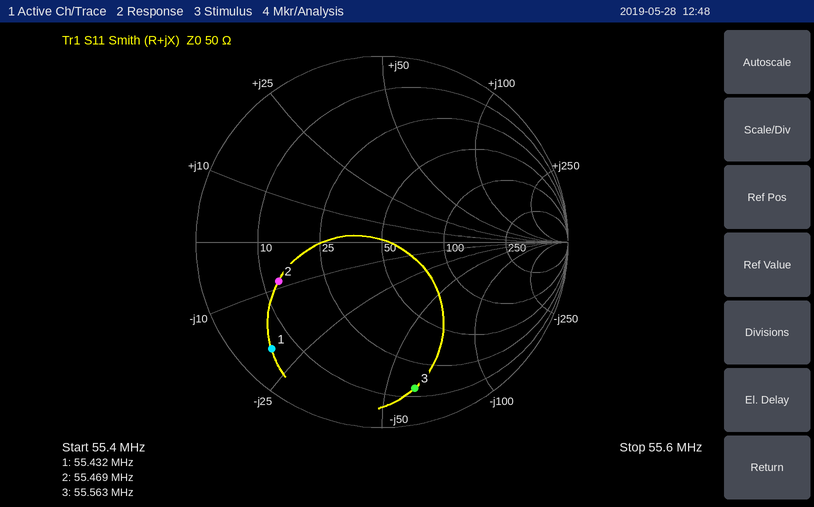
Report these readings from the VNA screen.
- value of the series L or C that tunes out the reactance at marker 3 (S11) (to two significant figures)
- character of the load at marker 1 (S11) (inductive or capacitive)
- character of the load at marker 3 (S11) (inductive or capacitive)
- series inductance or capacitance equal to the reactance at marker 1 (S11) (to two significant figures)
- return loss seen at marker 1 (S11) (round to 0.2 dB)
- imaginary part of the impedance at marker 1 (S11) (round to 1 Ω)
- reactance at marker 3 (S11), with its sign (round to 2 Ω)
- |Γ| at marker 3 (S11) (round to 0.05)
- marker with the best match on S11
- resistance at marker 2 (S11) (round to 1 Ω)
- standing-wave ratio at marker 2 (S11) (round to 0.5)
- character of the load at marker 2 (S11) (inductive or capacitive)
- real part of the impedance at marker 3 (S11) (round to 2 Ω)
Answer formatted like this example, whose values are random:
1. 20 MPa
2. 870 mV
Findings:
1. 170 nH
2. capacitive
3. capacitive
4. 140 pF
5. 1.6 dB
6. -20 Ω
7. -60 Ω
8. 0.80
9. marker 2
10. 13 Ω
11. 4.0
12. capacitive
13. 14 Ω
